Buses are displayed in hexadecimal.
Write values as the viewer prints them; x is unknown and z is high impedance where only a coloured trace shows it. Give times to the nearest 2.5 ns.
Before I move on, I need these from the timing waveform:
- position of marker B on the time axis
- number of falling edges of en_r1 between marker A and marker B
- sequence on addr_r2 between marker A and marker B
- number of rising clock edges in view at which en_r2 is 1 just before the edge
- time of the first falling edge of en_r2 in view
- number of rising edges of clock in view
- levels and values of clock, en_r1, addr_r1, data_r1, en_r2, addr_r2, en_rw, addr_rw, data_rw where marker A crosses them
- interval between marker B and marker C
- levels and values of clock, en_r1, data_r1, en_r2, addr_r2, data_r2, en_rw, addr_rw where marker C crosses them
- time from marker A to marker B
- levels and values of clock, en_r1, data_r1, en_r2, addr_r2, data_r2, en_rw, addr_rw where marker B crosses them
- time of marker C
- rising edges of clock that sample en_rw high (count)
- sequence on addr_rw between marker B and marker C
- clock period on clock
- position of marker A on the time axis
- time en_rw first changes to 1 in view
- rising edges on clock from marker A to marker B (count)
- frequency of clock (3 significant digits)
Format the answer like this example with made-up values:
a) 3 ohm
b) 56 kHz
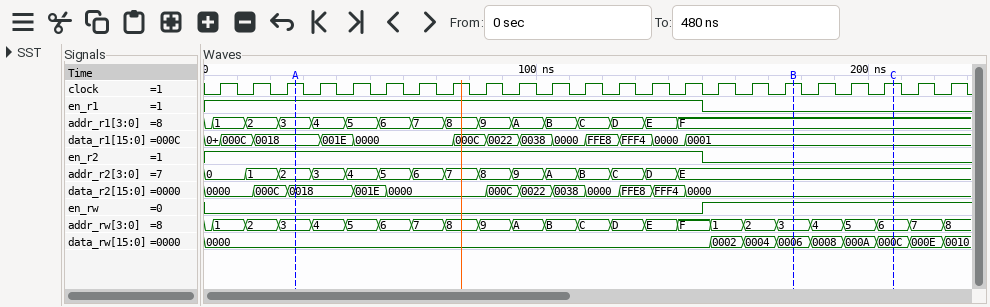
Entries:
a) 177.5 ns
b) 1
c) 2, 3, 4, 5, 6, 7, 8, 9, A, B, C, D, E
d) 15
e) 150 ns
f) 23
g) clock=1, en_r1=1, addr_r1=3, data_r1=0018, en_r2=1, addr_r2=2, en_rw=0, addr_rw=3, data_rw=0000
h) 30 ns
i) clock=1, en_r1=0, data_r1=0001, en_r2=0, addr_r2=E, data_r2=0000, en_rw=1, addr_rw=6
j) 150 ns
k) clock=1, en_r1=0, data_r1=0001, en_r2=0, addr_r2=E, data_r2=0000, en_rw=1, addr_rw=3
l) 207.5 ns
m) 8
n) 3, 4, 5, 6
o) 10 ns
p) 27.5 ns
q) 150 ns
r) 15
s) 100 MHz
